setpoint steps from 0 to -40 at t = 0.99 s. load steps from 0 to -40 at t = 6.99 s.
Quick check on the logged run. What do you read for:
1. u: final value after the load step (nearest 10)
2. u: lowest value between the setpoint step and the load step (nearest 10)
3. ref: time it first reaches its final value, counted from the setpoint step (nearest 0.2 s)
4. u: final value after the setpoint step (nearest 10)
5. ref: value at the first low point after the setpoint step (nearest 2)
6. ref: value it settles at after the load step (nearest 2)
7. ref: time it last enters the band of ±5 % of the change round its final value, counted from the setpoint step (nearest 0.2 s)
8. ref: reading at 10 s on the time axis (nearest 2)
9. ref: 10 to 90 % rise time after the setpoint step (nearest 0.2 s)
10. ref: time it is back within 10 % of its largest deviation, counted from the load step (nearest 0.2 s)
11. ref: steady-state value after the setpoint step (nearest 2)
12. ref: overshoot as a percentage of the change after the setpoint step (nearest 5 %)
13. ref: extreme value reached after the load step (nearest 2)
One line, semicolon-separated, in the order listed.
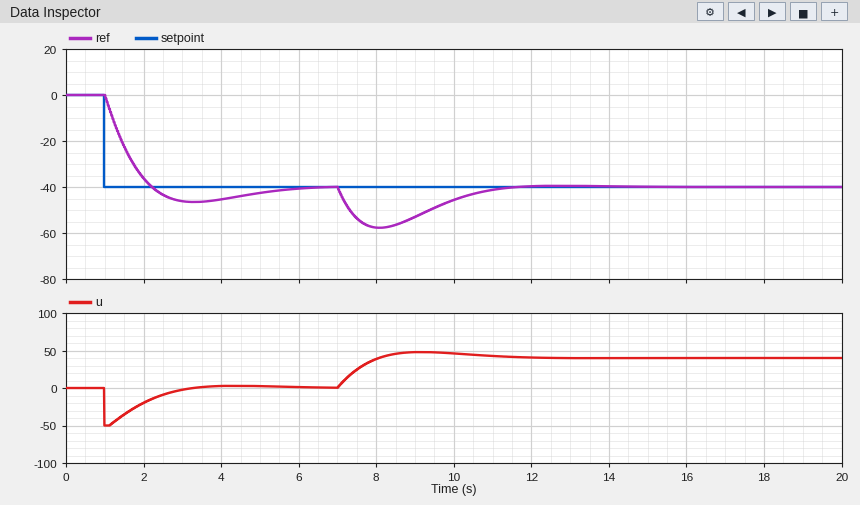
40; -50; 1.2 s; 0; -46; -40; 4.2 s; -46; 1.0 s; 3.8 s; -40; 15 %; -58
